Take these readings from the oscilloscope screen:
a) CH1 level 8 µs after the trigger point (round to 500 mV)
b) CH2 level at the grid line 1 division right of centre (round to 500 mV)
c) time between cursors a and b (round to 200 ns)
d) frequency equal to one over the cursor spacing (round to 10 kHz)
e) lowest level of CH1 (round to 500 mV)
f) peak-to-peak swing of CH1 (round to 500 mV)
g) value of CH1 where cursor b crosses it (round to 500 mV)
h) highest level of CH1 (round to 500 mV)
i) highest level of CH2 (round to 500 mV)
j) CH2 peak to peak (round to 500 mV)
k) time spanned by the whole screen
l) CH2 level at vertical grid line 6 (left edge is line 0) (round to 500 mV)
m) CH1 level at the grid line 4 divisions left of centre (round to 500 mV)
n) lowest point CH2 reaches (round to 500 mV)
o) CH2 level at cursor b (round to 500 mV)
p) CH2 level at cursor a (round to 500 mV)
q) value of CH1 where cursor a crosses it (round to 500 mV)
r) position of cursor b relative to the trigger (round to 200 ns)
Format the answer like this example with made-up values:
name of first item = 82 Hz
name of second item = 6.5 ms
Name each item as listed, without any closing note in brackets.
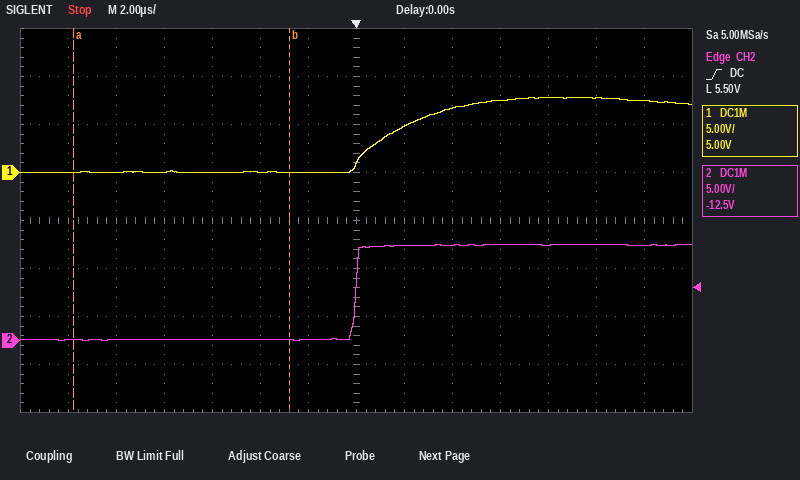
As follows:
CH1 level 8 µs after the trigger point = 8.0 V
CH2 level at the grid line 1 division right of centre = 10.0 V
time between cursors a and b = 9.0 µs
frequency equal to one over the cursor spacing = 110 kHz
lowest level of CH1 = 0.0 V
peak-to-peak swing of CH1 = 8.0 V
value of CH1 where cursor b crosses it = 0.0 V
highest level of CH1 = 8.0 V
highest level of CH2 = 10.0 V
CH2 peak to peak = 10.0 V
time spanned by the whole screen = 28 µs
CH2 level at vertical grid line 6 (left edge is line 0) = 0.0 V
CH1 level at the grid line 4 divisions left of centre = 0.0 V
lowest point CH2 reaches = 0.0 V
CH2 level at cursor b = 0.0 V
CH2 level at cursor a = 0.0 V
value of CH1 where cursor a crosses it = 0.0 V
position of cursor b relative to the trigger = -2.8 µs
